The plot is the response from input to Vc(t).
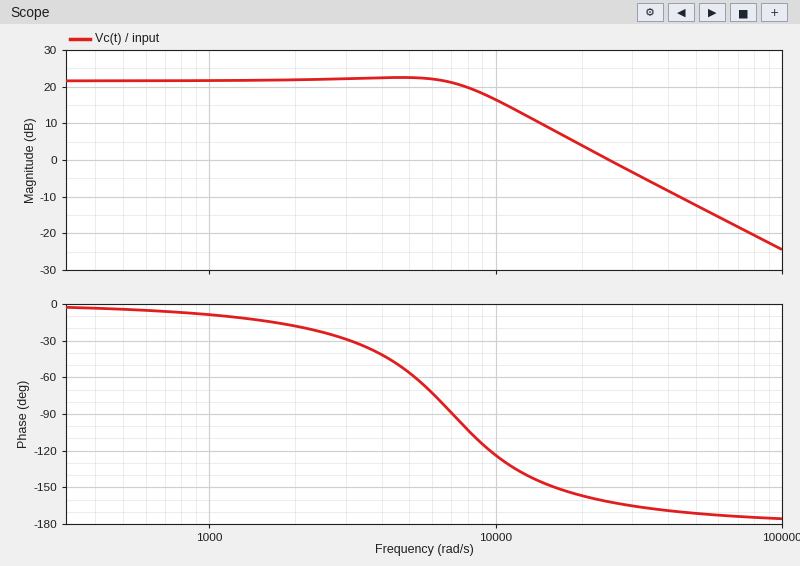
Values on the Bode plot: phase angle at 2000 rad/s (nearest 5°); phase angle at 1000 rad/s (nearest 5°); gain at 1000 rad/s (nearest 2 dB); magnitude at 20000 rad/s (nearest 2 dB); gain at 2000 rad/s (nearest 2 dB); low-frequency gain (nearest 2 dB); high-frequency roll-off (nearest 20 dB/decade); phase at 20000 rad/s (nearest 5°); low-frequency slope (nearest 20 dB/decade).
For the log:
-20°
-10°
22 dB
4 dB
22 dB
22 dB
-40 dB/decade
-155°
0 dB/decade
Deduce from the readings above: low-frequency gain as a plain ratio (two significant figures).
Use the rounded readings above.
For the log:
13
